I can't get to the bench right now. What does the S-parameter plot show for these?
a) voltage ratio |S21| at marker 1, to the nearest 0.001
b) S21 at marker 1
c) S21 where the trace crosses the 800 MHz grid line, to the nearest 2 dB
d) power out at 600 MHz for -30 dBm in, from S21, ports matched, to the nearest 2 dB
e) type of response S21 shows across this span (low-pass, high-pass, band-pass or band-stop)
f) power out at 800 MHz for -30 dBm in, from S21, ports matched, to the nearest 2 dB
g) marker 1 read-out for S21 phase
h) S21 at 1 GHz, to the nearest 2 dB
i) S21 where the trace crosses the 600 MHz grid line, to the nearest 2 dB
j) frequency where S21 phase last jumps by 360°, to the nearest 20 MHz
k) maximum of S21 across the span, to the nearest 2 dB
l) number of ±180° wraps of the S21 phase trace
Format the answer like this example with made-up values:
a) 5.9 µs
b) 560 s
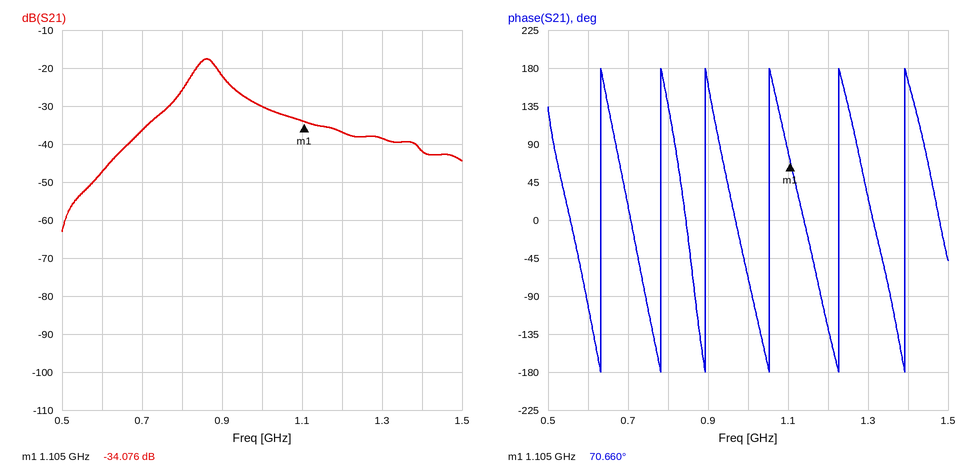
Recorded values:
a) 0.020
b) -34.076 dB
c) -26 dB
d) -78 dBm
e) band-pass
f) -56 dBm
g) 70.660°
h) -30 dB
i) -48 dB
j) 1.40 GHz
k) -18 dB
l) 6
